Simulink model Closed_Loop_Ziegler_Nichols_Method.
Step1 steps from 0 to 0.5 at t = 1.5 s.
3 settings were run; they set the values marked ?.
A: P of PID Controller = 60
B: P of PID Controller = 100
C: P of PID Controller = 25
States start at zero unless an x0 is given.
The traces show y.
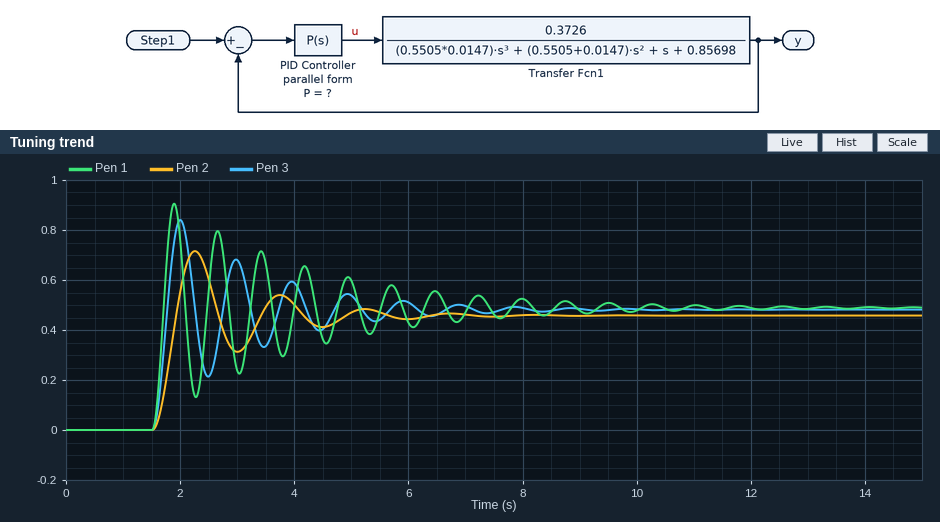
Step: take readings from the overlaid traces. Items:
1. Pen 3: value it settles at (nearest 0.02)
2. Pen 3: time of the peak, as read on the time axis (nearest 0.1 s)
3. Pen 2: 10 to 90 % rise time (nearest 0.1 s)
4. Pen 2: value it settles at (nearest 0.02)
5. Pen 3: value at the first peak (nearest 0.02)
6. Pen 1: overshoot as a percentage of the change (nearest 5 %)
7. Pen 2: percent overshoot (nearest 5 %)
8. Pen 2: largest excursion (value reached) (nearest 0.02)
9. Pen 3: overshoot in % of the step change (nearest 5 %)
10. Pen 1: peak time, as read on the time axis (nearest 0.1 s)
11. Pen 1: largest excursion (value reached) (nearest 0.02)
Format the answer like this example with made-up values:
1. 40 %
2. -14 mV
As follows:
1. 0.48
2. 2.0 s
3. 0.3 s
4. 0.46
5. 0.84
6. 85 %
7. 55 %
8. 0.72
9. 75 %
10. 1.9 s
11. 0.90
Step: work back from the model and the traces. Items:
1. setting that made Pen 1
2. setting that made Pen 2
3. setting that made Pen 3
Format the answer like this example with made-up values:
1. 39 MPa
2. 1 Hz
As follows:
1. B
2. C
3. A
